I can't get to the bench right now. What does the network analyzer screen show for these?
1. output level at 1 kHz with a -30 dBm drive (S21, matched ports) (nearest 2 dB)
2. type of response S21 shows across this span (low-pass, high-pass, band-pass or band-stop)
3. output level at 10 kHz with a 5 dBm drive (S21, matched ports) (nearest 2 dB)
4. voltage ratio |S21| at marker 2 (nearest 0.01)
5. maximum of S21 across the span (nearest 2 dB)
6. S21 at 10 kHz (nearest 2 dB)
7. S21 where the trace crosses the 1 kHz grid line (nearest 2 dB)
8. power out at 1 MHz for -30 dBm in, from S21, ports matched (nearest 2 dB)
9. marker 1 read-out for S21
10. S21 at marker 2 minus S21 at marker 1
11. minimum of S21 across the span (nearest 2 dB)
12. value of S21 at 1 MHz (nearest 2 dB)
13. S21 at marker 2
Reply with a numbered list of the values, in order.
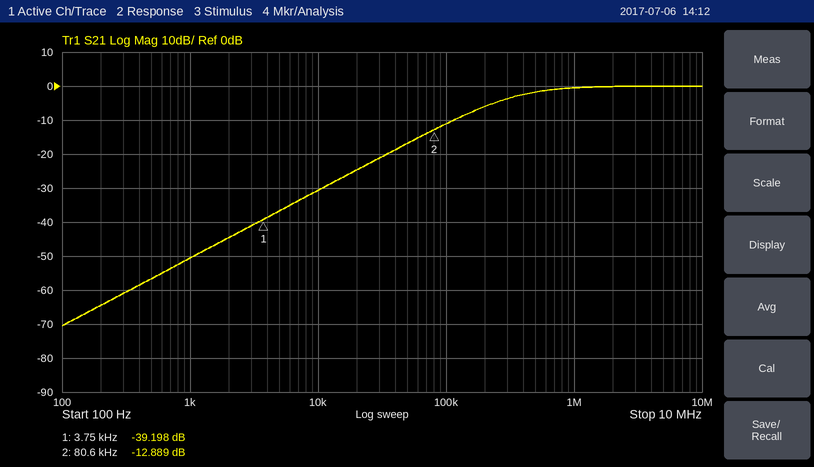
1. -80 dBm
2. high-pass
3. -26 dBm
4. 0.23
5. 0 dB
6. -30 dB
7. -50 dB
8. -30 dBm
9. -39.198 dB
10. 26.309 dB
11. -70 dB
12. 0 dB
13. -12.889 dB
